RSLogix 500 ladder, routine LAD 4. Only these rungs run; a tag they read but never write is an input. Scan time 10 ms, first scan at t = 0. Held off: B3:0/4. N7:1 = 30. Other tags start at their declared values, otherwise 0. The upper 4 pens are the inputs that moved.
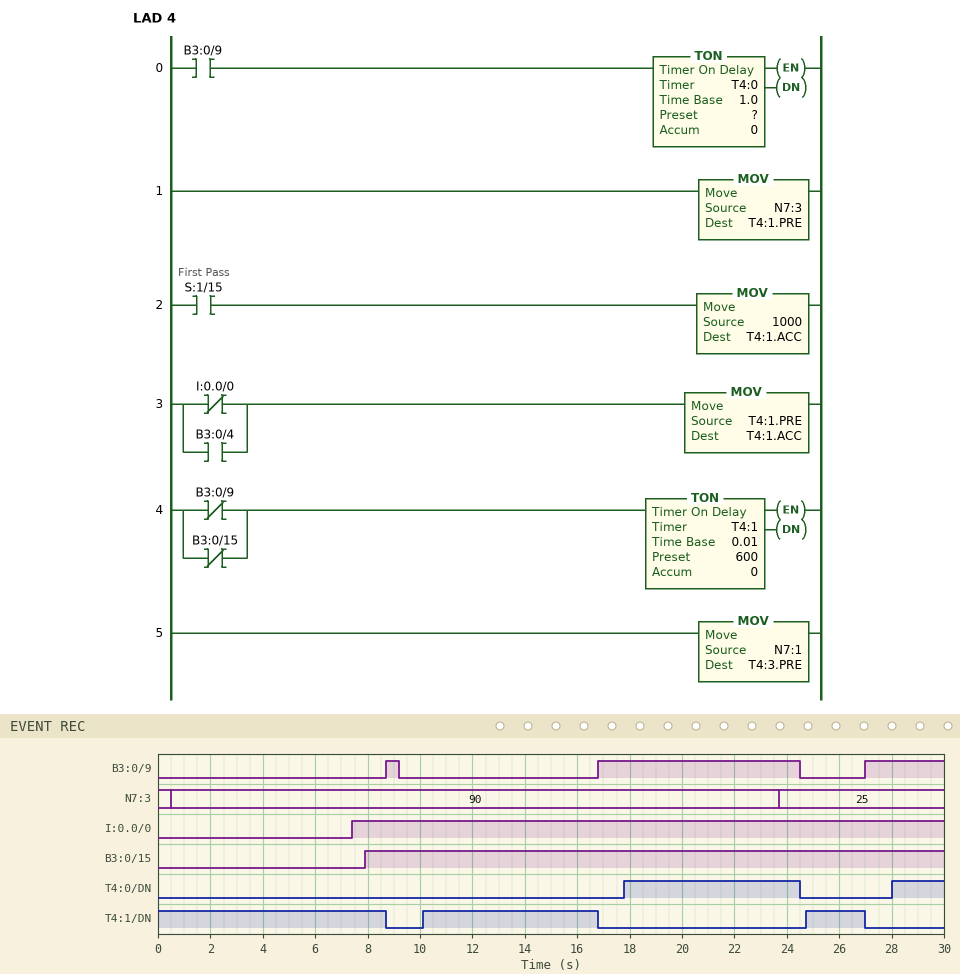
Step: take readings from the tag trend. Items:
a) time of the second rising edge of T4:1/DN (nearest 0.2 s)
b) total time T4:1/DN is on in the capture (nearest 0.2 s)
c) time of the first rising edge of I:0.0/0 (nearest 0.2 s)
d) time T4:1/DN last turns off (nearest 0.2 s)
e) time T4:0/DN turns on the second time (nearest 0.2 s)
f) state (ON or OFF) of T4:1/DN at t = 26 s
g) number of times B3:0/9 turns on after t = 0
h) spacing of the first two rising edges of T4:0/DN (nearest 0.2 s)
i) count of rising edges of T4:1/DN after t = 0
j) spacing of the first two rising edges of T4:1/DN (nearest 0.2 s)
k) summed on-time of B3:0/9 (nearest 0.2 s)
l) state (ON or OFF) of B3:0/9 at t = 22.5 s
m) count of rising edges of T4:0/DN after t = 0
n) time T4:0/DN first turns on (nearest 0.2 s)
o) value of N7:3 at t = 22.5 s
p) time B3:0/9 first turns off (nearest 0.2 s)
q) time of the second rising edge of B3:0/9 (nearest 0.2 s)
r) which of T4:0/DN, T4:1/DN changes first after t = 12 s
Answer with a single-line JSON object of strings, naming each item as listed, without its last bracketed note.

{"time of the second rising edge of T4:1/DN": "24.8 s", "total time T4:1/DN is on in the capture": "17.6 s", "time of the first rising edge of I:0.0/0": "7.4 s", "time T4:1/DN last turns off": "27.0 s", "time T4:0/DN turns on the second time": "28.0 s", "state (ON or OFF) of T4:1/DN at t = 26 s": "ON", "number of times B3:0/9 turns on after t = 0": "3", "spacing of the first two rising edges of T4:0/DN": "10.2 s", "count of rising edges of T4:1/DN after t = 0": "2", "spacing of the first two rising edges of T4:1/DN": "14.6 s", "summed on-time of B3:0/9": "11.2 s", "state (ON or OFF) of B3:0/9 at t = 22.5 s": "ON", "count of rising edges of T4:0/DN after t = 0": "2", "time T4:0/DN first turns on": "17.8 s", "value of N7:3 at t = 22.5 s": "90", "time B3:0/9 first turns off": "9.2 s", "time of the second rising edge of B3:0/9": "16.8 s", "which of T4:0/DN, T4:1/DN changes first after t = 12 s": "T4:1/DN"}
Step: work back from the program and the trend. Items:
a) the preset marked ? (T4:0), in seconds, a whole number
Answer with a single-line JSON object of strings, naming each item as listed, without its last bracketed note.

{"the preset marked ? (T4:0), in seconds, a whole number": "1 s"}
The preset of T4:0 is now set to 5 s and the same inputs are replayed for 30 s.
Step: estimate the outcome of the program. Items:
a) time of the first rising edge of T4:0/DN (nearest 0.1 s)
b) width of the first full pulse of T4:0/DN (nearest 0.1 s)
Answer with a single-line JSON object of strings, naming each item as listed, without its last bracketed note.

{"time of the first rising edge of T4:0/DN": "21.8 s", "width of the first full pulse of T4:0/DN": "2.7 s"}
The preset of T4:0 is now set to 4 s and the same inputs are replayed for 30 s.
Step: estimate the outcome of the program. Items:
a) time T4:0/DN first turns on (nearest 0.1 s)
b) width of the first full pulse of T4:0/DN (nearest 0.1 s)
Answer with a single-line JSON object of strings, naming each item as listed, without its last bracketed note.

{"time T4:0/DN first turns on": "20.8 s", "width of the first full pulse of T4:0/DN": "3.7 s"}
